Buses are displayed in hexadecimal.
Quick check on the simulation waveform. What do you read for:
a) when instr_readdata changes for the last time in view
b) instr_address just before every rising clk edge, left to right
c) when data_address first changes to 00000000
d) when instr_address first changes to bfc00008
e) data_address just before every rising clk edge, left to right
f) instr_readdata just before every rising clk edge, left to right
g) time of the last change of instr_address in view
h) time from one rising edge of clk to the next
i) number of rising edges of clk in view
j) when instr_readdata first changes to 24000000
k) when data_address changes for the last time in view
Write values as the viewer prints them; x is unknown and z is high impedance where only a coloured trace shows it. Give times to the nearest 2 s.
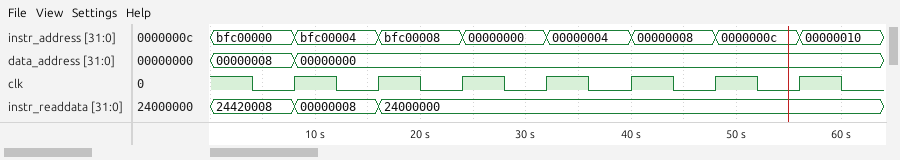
16 s
bfc00000, bfc00004, bfc00008, 00000000, 00000004, 00000008, 0000000c
8 s
16 s
00000008, 00000000, 00000000, 00000000, 00000000, 00000000, 00000000
24420008, 00000008, 24000000, 24000000, 24000000, 24000000, 24000000
56 s
8 s
7
16 s
8 s
